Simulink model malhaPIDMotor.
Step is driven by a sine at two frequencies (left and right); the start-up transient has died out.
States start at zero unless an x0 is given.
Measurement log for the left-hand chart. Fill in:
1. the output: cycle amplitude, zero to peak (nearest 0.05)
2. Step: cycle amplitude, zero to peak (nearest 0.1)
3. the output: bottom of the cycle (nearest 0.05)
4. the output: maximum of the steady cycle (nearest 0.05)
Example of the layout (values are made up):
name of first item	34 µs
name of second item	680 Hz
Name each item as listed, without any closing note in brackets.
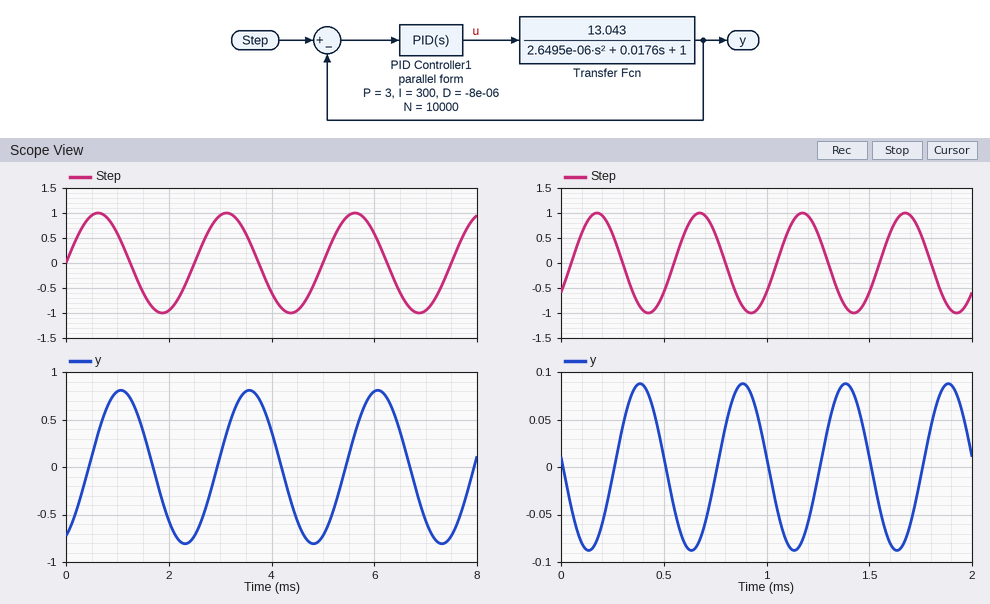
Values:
the output: cycle amplitude, zero to peak	0.80
Step: cycle amplitude, zero to peak	1.0
the output: bottom of the cycle	-0.80
the output: maximum of the steady cycle	0.80
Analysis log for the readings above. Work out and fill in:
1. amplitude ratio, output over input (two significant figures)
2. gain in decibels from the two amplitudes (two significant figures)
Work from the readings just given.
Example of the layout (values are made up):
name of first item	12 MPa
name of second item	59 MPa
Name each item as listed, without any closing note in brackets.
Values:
amplitude ratio, output over input	0.80
gain in decibels from the two amplitudes	-1.9 dB
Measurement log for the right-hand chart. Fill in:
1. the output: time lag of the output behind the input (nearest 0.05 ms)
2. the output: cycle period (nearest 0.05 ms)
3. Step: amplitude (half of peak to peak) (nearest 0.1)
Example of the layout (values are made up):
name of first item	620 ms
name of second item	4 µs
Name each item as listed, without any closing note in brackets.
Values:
the output: time lag of the output behind the input	0.20 ms
the output: cycle period	0.50 ms
Step: amplitude (half of peak to peak)	1.0
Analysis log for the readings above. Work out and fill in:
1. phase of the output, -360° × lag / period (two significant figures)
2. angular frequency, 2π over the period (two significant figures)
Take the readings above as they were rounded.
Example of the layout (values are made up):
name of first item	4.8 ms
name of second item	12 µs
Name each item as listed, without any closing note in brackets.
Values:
phase of the output, -360° × lag / period	-140°
angular frequency, 2π over the period	13 rad/ms
